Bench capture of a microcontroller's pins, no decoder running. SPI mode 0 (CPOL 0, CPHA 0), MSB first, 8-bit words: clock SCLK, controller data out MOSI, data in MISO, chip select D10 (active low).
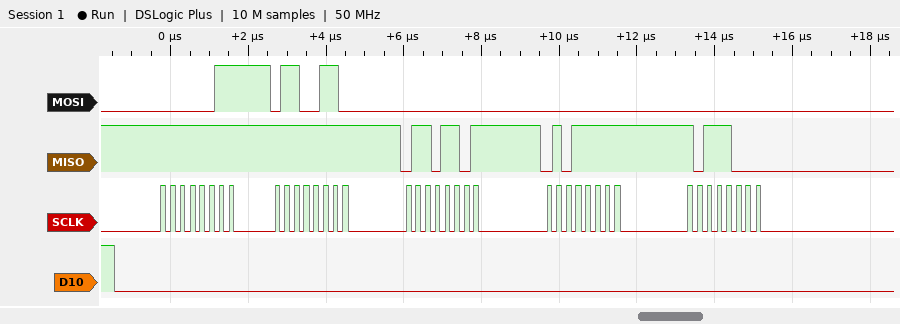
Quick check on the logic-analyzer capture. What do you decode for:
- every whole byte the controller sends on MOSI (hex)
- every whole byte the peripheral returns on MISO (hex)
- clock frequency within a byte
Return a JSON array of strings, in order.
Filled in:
["03 66 00 00 00", "FF FF 6D 5F B8", "4 MHz"]
